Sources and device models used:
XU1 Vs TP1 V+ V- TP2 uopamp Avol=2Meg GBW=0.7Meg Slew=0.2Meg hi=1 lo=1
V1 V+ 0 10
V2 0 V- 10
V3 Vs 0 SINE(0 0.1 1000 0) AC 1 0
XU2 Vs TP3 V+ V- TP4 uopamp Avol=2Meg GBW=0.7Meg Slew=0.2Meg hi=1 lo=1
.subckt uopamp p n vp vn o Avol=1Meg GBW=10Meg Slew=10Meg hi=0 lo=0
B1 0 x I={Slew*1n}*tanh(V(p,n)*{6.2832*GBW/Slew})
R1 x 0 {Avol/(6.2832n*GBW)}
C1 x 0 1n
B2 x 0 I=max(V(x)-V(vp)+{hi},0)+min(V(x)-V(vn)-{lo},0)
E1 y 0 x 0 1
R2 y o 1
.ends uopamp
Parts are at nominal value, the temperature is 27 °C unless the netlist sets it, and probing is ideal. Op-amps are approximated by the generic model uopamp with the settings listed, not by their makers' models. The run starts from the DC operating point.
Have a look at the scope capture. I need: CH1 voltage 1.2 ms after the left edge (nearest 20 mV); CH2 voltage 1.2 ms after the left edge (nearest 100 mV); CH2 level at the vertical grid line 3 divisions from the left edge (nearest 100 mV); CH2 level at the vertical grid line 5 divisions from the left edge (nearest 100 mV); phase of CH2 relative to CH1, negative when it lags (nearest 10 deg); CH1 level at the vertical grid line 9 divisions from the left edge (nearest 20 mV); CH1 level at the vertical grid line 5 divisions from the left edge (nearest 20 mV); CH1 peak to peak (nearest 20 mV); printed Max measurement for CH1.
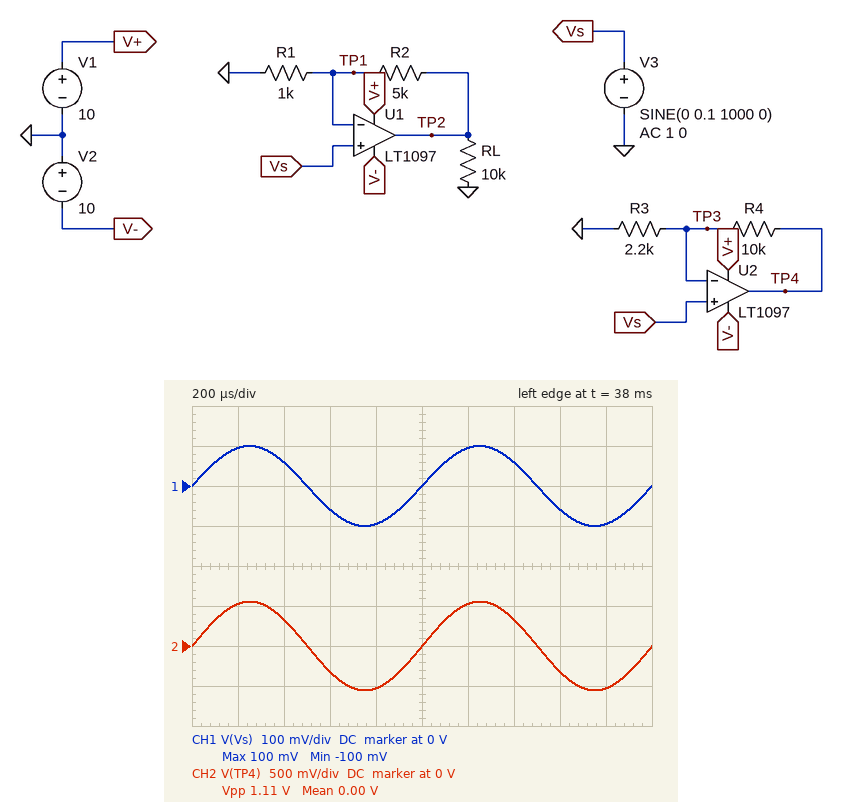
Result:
100 mV
500 mV
-300 mV
0 V
0 deg
-100 mV
0 V
200 mV
100 mV
